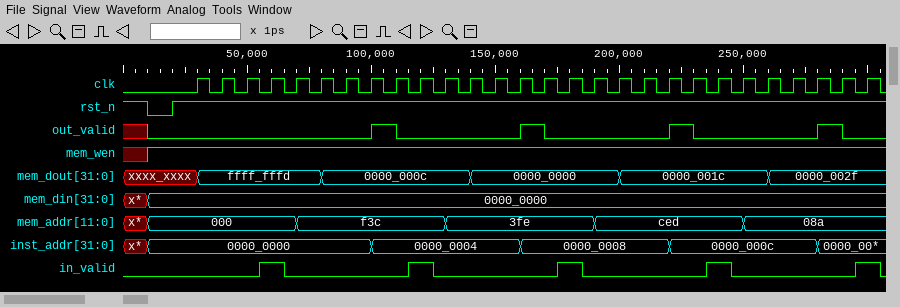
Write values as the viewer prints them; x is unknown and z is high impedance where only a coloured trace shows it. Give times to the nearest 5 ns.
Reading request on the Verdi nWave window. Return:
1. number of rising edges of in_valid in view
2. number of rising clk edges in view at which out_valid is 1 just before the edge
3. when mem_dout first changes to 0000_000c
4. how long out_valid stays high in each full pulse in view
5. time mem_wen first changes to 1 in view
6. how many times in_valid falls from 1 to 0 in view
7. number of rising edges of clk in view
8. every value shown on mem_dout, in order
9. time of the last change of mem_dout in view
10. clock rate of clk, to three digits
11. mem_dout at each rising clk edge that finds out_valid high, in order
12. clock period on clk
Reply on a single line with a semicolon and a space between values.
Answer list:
5; 4; 80 ns; 10 ns, 10 ns, 10 ns, 10 ns; 10 ns; 5; 28; xxxx_xxxx, ffff_fffd, 0000_000c, 0000_0000, 0000_001c, 0000_002f; 260 ns; 100 MHz; 0000_000c, 0000_0000, 0000_001c, 0000_002f; 10 ns
